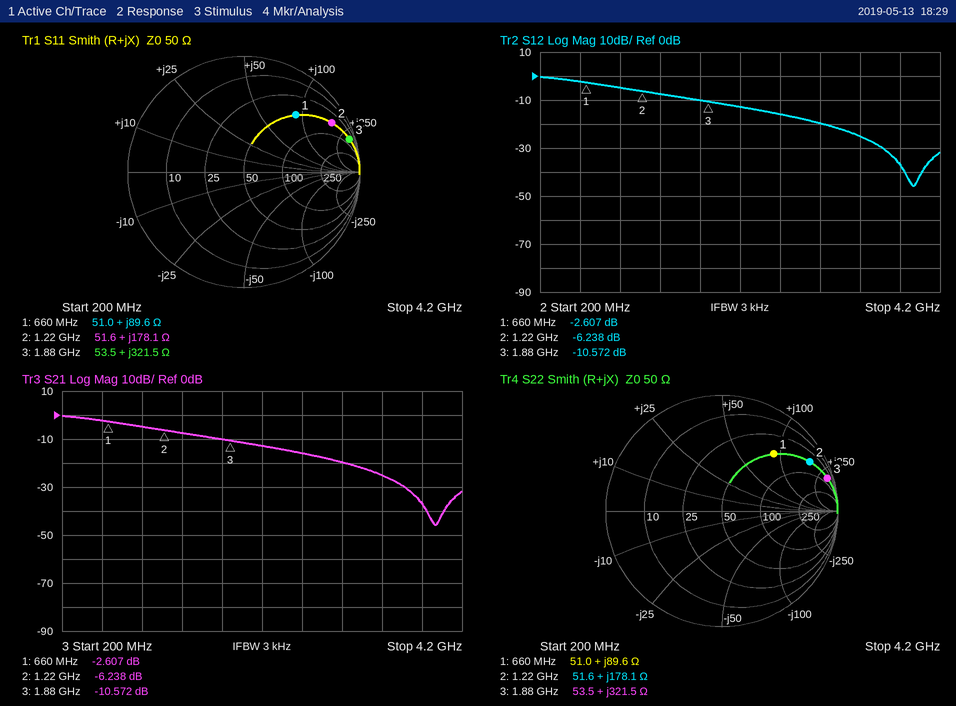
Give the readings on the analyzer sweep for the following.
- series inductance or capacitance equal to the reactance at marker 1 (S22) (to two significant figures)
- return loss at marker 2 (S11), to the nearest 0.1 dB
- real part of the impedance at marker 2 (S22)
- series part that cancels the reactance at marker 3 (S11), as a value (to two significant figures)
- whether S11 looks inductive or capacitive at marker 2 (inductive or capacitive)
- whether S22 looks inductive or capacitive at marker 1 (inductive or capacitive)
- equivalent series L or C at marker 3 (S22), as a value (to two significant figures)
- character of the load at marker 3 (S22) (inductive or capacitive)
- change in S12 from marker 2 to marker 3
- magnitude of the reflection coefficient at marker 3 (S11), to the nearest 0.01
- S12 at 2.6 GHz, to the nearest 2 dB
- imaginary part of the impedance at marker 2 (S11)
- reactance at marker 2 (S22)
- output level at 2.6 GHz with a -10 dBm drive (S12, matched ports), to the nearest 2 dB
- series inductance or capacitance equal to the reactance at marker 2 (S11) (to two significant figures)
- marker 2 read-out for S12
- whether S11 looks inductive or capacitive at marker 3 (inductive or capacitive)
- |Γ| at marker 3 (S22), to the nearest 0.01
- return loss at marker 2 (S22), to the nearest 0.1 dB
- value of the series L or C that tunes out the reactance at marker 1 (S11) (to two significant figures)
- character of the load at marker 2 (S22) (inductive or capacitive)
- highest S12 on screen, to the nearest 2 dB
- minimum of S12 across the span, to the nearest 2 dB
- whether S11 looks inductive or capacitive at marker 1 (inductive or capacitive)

22 nH
1.2 dB
51.6 Ω
260 fF
inductive
inductive
27 nH
inductive
-4.334 dB
0.95
-16 dB
+178.1 Ω
+178.1 Ω
-26 dBm
23 nH
-6.238 dB
inductive
0.95
1.2 dB
2.7 pF
inductive
0 dB
-46 dB
inductive
